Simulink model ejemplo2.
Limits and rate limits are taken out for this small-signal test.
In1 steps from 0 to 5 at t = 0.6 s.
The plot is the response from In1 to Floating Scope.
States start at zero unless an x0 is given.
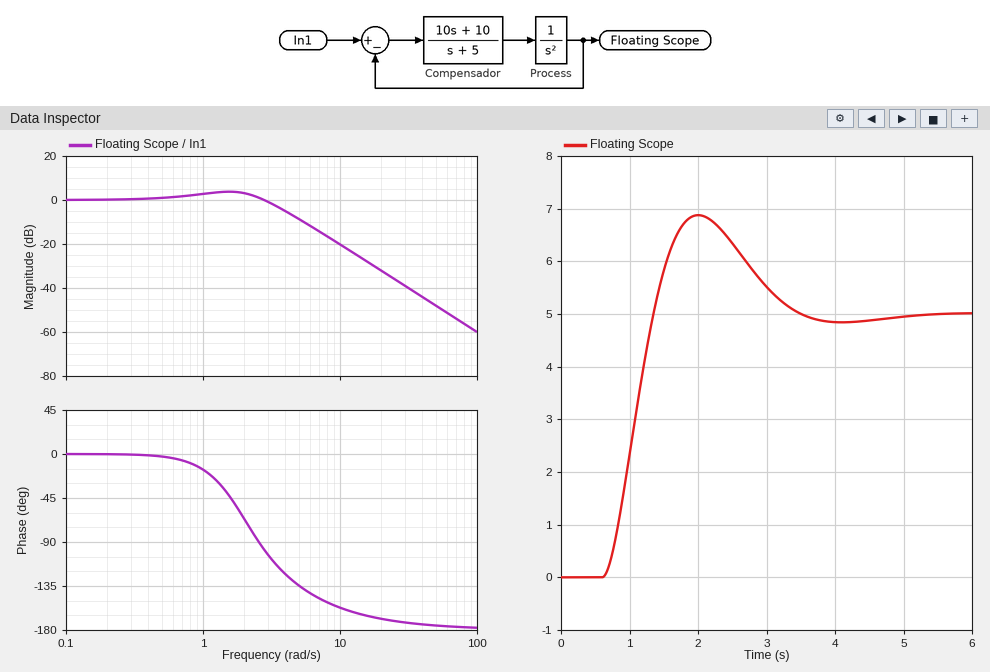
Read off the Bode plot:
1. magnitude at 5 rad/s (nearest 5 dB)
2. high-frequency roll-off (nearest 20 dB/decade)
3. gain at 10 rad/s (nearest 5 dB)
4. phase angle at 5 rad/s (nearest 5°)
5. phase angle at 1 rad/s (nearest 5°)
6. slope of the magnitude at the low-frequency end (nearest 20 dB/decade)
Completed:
-10 dB
-40 dB/decade
-20 dB
-135°
-15°
0 dB/decade
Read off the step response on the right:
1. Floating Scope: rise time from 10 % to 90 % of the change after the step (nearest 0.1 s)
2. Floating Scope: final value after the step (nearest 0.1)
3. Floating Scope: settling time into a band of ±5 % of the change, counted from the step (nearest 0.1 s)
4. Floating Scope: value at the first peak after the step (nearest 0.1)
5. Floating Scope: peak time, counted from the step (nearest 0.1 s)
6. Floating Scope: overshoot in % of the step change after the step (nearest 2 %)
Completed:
0.5 s
5.0
2.6 s
6.9
1.4 s
38 %
